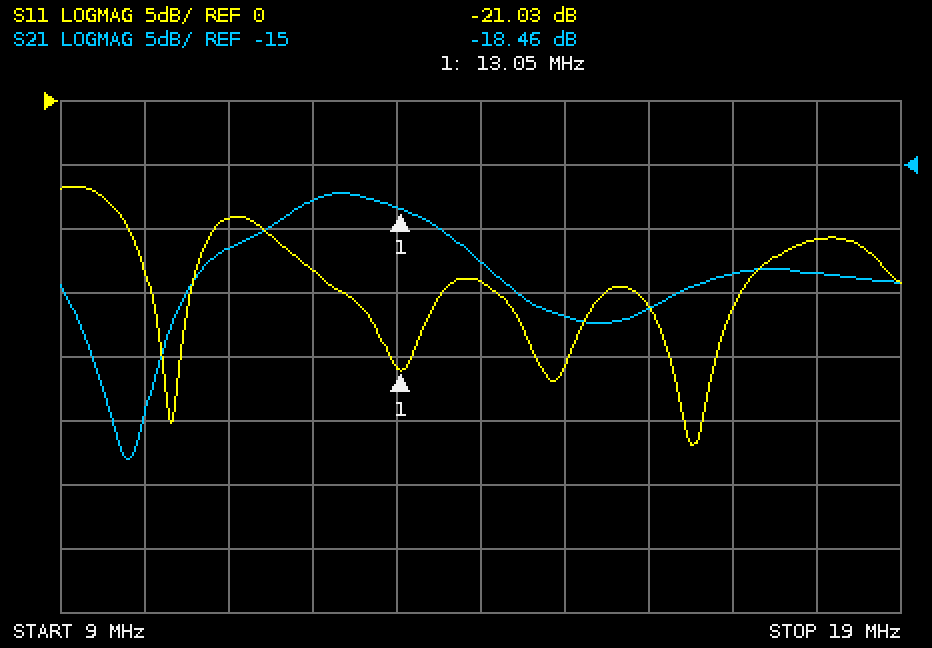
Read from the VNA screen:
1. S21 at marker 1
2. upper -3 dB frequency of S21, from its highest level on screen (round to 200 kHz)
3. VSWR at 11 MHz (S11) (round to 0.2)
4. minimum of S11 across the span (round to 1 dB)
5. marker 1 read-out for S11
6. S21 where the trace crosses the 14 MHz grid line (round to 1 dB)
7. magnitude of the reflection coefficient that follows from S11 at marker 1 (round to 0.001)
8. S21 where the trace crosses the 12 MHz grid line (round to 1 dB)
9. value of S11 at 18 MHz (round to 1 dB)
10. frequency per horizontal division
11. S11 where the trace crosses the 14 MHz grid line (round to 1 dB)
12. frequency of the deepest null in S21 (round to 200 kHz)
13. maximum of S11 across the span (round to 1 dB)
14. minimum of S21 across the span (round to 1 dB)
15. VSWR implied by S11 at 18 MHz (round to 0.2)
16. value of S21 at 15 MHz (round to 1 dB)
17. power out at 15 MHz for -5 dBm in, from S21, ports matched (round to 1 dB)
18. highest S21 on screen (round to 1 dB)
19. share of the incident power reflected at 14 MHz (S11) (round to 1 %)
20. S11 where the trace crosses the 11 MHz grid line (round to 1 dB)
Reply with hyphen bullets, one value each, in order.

- -18.46 dB
- 13.6 MHz
- 2.0
- -27 dB
- -21.03 dB
- -23 dB
- 0.089
- -18 dB
- -11 dB
- 1 MHz
- -14 dB
- 9.8 MHz
- -7 dB
- -38 dB
- 1.8
- -27 dB
- -32 dBm
- -17 dB
- 4 %
- -9 dB
